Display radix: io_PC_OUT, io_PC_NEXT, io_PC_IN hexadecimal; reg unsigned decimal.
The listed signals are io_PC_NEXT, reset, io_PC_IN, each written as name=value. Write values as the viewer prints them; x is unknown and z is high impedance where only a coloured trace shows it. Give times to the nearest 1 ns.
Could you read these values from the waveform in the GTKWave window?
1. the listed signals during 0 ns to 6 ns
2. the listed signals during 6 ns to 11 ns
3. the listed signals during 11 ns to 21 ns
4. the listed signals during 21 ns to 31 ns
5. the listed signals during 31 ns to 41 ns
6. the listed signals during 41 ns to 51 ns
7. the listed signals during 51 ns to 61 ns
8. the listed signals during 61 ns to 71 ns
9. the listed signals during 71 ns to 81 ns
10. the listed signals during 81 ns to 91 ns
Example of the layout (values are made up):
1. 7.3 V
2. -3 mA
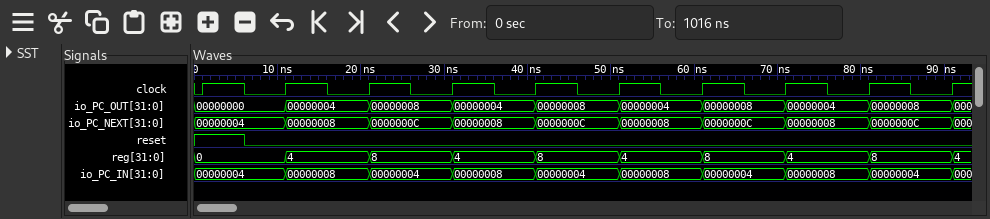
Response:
1. io_PC_NEXT=00000004, reset=1, io_PC_IN=00000004
2. io_PC_NEXT=00000004, reset=0, io_PC_IN=00000004
3. io_PC_NEXT=00000008, reset=0, io_PC_IN=00000008
4. io_PC_NEXT=0000000C, reset=0, io_PC_IN=00000004
5. io_PC_NEXT=00000008, reset=0, io_PC_IN=00000008
6. io_PC_NEXT=0000000C, reset=0, io_PC_IN=00000004
7. io_PC_NEXT=00000008, reset=0, io_PC_IN=00000008
8. io_PC_NEXT=0000000C, reset=0, io_PC_IN=00000004
9. io_PC_NEXT=00000008, reset=0, io_PC_IN=00000008
10. io_PC_NEXT=0000000C, reset=0, io_PC_IN=00000004
